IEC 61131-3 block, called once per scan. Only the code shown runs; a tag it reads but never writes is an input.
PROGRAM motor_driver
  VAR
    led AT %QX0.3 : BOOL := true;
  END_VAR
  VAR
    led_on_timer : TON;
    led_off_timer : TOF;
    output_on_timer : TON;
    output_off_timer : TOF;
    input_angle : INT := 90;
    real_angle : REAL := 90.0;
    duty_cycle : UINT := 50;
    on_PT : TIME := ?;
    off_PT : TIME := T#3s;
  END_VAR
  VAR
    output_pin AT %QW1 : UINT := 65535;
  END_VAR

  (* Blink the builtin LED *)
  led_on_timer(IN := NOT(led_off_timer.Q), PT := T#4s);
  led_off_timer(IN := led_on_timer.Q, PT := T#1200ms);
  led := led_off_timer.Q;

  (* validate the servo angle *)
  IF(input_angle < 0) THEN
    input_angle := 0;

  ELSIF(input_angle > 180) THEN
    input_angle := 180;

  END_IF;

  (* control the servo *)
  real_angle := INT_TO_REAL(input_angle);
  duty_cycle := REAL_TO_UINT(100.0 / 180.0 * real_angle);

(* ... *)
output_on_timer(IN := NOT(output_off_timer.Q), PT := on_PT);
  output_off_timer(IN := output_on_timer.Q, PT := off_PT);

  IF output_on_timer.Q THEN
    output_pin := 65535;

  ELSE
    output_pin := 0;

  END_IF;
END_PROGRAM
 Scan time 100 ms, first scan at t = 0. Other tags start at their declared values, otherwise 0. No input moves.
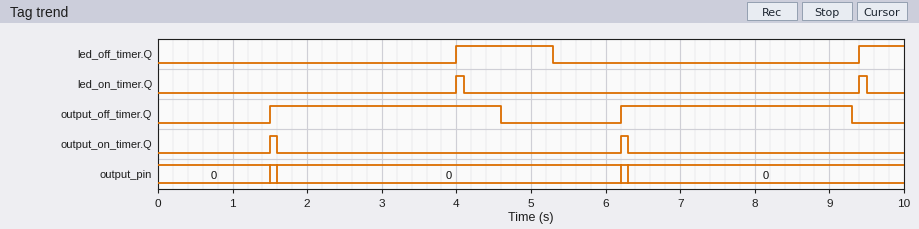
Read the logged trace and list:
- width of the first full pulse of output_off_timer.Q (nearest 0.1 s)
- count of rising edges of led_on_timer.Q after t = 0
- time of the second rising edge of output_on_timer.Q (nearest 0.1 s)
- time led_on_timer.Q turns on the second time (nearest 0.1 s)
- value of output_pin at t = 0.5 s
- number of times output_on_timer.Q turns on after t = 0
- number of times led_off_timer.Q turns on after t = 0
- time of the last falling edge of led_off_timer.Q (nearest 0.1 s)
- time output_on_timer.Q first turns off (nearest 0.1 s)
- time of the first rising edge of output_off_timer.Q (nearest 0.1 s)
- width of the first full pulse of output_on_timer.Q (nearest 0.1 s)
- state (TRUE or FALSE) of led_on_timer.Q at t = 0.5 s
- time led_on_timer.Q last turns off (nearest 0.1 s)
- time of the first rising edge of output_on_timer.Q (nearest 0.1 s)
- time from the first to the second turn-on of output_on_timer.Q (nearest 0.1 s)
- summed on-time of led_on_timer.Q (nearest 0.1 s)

3.1 s
2
6.2 s
9.4 s
0
2
2
5.3 s
1.6 s
1.5 s
0.1 s
FALSE
9.5 s
1.5 s
4.7 s
0.2 s
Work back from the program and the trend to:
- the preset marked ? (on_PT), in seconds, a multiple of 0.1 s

1.5 s
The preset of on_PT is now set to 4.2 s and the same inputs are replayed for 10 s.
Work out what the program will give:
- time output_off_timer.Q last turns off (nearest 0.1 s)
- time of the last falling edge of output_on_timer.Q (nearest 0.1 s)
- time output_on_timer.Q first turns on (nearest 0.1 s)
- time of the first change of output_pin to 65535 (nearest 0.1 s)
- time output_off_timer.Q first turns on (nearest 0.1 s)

7.3 s
4.3 s
4.2 s
4.2 s
4.2 s
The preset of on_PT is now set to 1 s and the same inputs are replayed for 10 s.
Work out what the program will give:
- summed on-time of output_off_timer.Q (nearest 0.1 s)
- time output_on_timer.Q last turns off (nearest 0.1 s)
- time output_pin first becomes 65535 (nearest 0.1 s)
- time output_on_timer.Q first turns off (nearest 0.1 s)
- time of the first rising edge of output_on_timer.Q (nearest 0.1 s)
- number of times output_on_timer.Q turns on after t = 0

6.8 s
9.5 s
1.0 s
1.1 s
1.0 s
3
